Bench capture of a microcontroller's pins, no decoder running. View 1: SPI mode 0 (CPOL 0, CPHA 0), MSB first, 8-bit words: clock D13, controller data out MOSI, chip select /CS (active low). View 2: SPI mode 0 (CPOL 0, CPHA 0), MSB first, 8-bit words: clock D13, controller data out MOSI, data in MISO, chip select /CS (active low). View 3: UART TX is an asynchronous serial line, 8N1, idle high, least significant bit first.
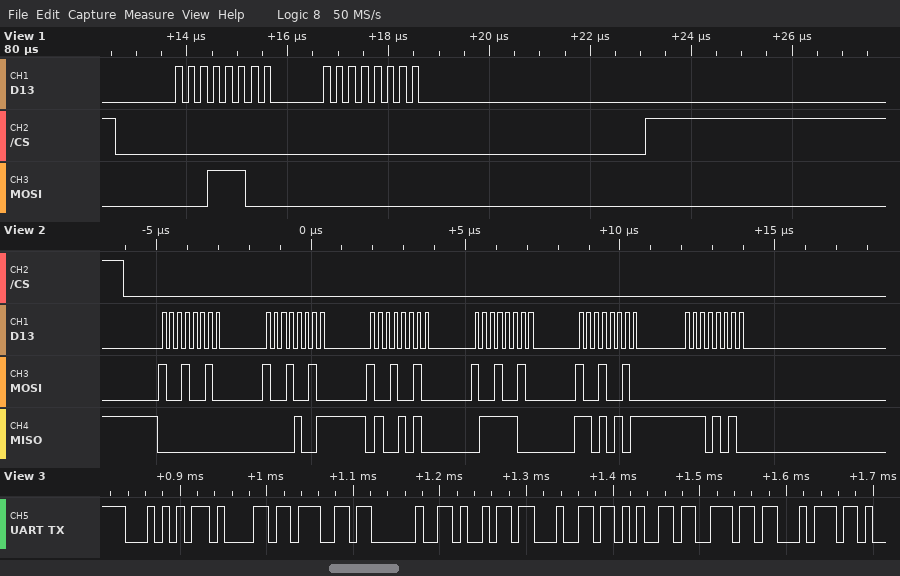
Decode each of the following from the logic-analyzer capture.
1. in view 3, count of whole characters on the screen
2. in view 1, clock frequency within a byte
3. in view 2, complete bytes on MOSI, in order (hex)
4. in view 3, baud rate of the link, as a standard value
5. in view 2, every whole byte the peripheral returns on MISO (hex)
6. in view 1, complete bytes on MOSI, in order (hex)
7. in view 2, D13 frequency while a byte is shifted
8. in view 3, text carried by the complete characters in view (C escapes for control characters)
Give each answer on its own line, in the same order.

9
4 MHz
92 92 92 92 92 00
115200 baud
00 09 4A 7C D5 EA
0x1C 0x00
4 MHz
"Tag ident"
